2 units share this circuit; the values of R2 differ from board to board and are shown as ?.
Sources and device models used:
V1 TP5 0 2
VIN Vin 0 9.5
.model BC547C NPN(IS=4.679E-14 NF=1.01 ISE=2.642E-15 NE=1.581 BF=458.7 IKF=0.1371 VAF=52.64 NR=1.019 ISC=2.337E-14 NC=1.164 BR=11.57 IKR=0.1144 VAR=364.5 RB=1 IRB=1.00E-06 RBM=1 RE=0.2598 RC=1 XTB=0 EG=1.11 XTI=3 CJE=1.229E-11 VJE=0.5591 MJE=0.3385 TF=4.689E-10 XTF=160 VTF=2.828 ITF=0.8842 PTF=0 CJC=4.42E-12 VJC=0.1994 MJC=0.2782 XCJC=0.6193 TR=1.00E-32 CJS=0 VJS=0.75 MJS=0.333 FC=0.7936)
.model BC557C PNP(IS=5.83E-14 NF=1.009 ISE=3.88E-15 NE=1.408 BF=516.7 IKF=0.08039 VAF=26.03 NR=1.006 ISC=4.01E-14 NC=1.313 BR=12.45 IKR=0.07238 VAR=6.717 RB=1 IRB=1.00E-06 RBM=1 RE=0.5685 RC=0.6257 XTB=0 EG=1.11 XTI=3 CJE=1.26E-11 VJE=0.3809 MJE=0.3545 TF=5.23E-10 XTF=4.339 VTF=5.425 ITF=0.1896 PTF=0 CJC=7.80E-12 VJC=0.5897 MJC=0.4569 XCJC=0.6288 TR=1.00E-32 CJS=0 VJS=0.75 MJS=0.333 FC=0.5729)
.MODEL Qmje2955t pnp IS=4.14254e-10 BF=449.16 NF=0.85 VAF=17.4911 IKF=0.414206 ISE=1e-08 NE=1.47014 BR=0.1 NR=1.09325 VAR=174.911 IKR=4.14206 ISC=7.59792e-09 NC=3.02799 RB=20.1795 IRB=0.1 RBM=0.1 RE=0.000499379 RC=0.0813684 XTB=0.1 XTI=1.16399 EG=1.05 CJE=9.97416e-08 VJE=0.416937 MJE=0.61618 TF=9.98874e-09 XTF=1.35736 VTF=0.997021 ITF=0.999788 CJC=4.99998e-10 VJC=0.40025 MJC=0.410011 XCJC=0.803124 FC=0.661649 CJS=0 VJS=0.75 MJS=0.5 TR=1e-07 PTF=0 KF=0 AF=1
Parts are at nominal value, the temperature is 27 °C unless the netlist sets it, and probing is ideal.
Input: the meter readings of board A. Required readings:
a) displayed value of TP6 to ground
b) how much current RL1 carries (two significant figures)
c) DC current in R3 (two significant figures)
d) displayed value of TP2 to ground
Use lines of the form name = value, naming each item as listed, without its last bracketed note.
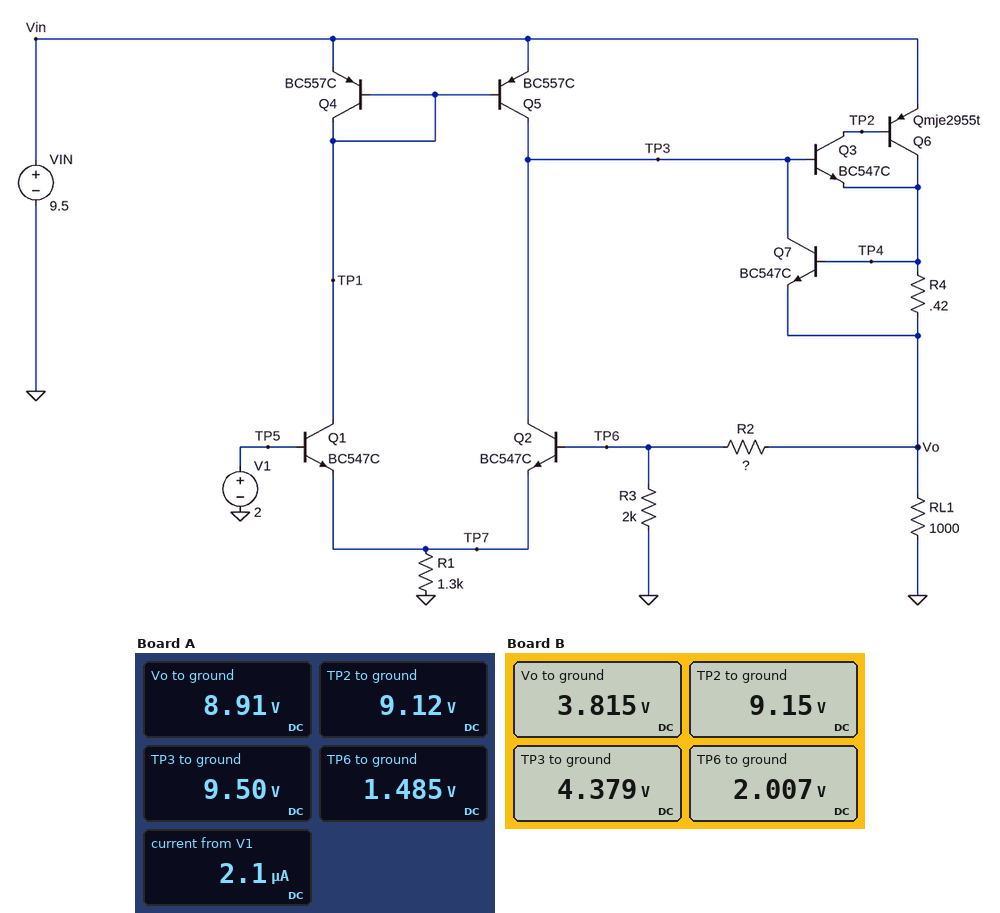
displayed value of TP6 to ground = 1.485 V
how much current RL1 carries = 8.9 mA
DC current in R3 = 740 µA
displayed value of TP2 to ground = 9.12 V
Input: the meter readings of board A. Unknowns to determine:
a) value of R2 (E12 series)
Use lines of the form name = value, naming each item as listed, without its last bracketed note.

value of R2 = 10 kΩ
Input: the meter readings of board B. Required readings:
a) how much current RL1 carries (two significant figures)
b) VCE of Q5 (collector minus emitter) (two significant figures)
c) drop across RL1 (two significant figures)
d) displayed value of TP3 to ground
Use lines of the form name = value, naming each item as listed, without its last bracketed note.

how much current RL1 carries = 3.8 mA
VCE of Q5 (collector minus emitter) = -5.1 V
drop across RL1 = 3.8 V
displayed value of TP3 to ground = 4.379 V
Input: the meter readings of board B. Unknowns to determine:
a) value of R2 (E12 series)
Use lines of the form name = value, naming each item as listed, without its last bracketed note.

value of R2 = 1.8 kΩ
